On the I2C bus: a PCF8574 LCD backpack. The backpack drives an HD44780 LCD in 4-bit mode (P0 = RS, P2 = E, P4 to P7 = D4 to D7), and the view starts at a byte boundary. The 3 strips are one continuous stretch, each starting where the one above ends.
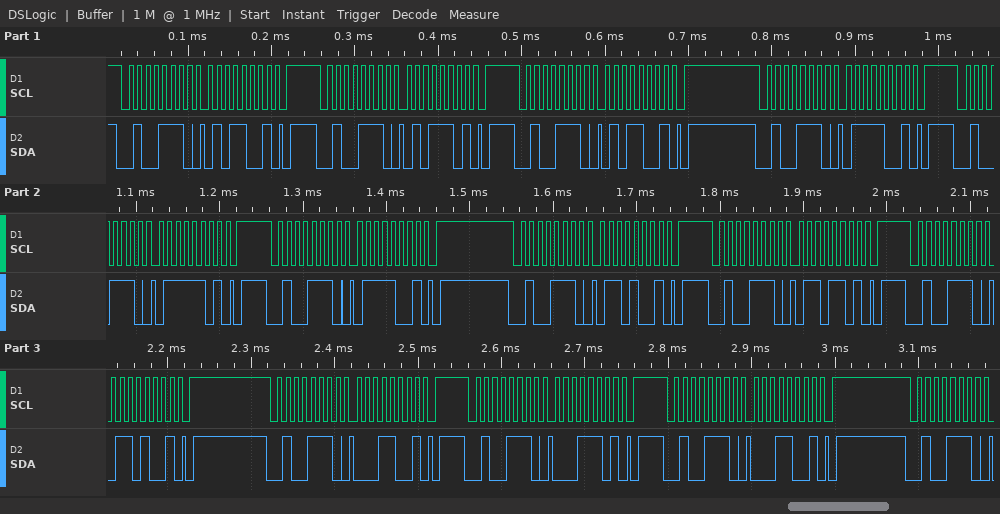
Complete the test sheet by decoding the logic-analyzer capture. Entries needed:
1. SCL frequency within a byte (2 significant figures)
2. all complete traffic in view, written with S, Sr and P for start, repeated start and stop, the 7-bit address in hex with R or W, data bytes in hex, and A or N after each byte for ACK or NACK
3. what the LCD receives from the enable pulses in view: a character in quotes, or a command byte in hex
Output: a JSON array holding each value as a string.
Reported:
["100 kHz", "S 27W A 59 A P S 27W A 5D A P S 27W A 59 A P S 27W A 79 A P S 27W A 7D A P S 27W A 79 A P S 27W A 69 A P S 27W A 6D A P S 27W A 69 A P S 27W A 19 A P S 27W A 1D A P S 27W A 19 A P S 27W A", "'W' 'a'"]
